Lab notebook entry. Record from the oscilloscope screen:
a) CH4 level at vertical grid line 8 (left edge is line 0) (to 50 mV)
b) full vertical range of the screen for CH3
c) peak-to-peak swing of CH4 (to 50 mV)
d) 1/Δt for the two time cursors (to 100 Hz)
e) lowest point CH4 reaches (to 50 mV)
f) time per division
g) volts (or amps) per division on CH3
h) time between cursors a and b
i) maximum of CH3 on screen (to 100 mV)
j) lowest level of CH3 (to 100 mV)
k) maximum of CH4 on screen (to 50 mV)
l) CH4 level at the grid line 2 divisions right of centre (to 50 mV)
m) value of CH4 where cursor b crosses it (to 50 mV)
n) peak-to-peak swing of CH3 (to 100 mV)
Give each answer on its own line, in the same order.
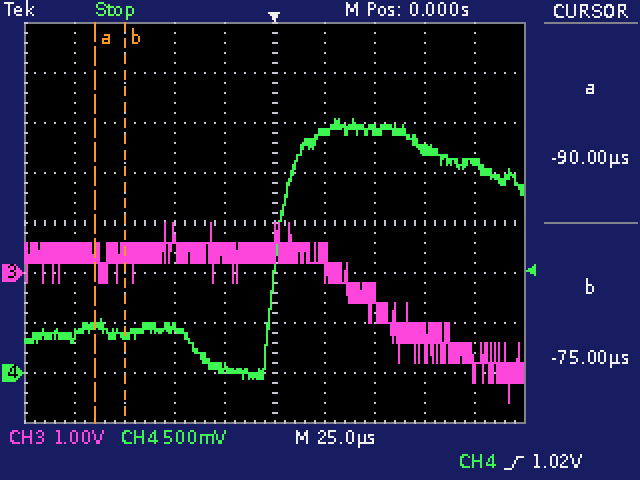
2.25 V
8 V
2.60 V
66.7 kHz
-50 mV
25 µs
1 V
15.0 µs
1.0 V
-2.6 V
2.55 V
2.45 V
400 mV
3.6 V
